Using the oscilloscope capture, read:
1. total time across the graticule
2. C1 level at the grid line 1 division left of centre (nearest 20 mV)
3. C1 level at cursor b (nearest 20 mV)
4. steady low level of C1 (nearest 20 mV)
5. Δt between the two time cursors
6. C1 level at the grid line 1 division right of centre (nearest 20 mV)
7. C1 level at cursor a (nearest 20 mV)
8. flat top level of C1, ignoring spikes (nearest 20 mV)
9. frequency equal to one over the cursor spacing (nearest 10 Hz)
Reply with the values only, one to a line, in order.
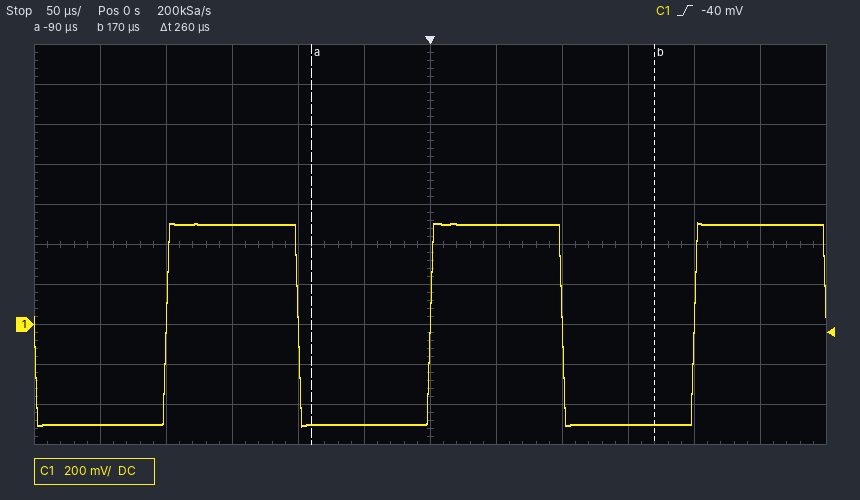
600 µs
-500 mV
-500 mV
-500 mV
260 µs
500 mV
-500 mV
500 mV
3.85 kHz
